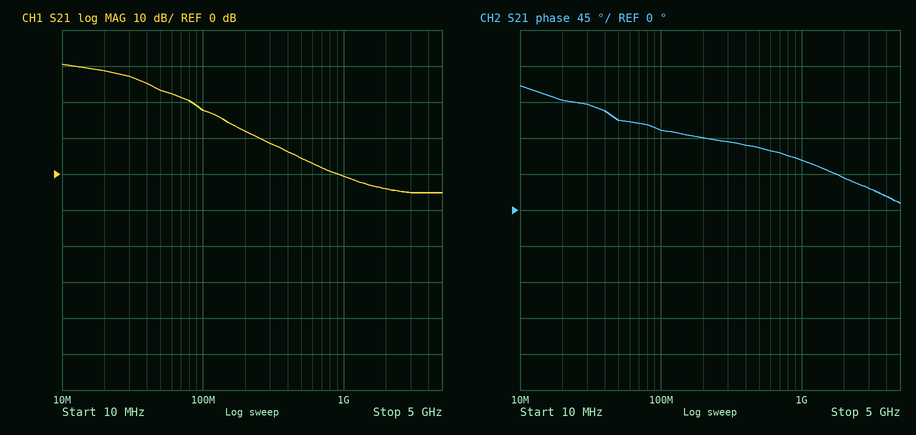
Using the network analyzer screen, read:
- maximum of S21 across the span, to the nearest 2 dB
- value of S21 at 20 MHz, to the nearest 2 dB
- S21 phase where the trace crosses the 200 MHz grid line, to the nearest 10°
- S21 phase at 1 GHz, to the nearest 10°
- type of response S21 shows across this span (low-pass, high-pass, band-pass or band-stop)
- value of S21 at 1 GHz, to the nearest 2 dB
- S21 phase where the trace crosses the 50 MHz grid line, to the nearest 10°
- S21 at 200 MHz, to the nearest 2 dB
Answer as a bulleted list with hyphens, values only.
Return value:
- 30 dB
- 28 dB
- 90°
- 60°
- low-pass
- 0 dB
- 110°
- 12 dB
